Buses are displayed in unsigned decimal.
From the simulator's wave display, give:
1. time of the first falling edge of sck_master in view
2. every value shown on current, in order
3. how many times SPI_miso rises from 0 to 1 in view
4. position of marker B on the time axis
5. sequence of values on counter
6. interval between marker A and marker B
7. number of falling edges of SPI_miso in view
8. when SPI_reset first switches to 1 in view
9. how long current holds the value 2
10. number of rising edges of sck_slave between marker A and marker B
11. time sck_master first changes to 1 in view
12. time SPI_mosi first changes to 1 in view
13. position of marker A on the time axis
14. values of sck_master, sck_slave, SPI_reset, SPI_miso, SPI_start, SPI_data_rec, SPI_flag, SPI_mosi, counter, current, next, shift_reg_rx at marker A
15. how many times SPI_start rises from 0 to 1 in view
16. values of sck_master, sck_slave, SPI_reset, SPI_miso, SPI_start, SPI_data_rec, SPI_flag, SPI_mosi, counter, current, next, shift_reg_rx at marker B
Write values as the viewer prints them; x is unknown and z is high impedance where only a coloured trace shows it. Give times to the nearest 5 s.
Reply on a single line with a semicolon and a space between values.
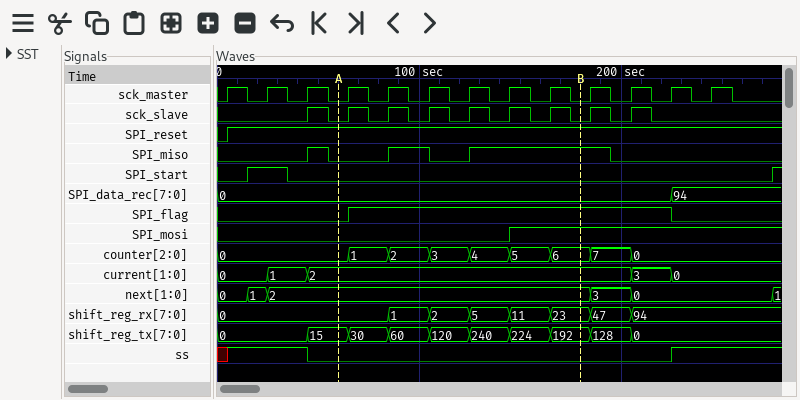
15 s; 0, 1, 2, 3, 0; 3; 180 s; 0, 1, 2, 3, 4, 5, 6, 7, 0; 120 s; 3; 5 s; 160 s; 6; 5 s; 145 s; 60 s; sck_master=0, sck_slave=0, SPI_reset=1, SPI_miso=0, SPI_start=0, SPI_data_rec=0, SPI_flag=0, SPI_mosi=0, counter=0, current=2, next=2, shift_reg_rx=0; 2; sck_master=0, sck_slave=0, SPI_reset=1, SPI_miso=1, SPI_start=0, SPI_data_rec=0, SPI_flag=1, SPI_mosi=1, counter=6, current=2, next=2, shift_reg_rx=23
